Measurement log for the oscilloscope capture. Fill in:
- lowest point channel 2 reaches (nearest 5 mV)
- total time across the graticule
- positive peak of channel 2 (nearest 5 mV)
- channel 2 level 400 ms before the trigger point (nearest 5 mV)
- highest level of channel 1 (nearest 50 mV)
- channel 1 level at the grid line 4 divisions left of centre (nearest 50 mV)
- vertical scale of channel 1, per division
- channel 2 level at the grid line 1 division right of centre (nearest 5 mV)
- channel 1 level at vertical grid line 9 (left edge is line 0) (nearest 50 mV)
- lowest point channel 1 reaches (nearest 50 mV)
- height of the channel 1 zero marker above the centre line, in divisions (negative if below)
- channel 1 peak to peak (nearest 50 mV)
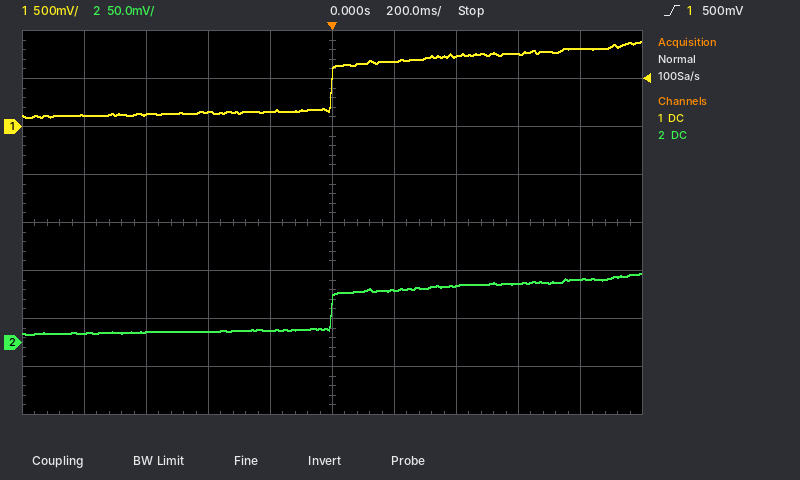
10 mV
2 s
70 mV
10 mV
900 mV
100 mV
500 mV
55 mV
800 mV
100 mV
+2.0 div
800 mV
